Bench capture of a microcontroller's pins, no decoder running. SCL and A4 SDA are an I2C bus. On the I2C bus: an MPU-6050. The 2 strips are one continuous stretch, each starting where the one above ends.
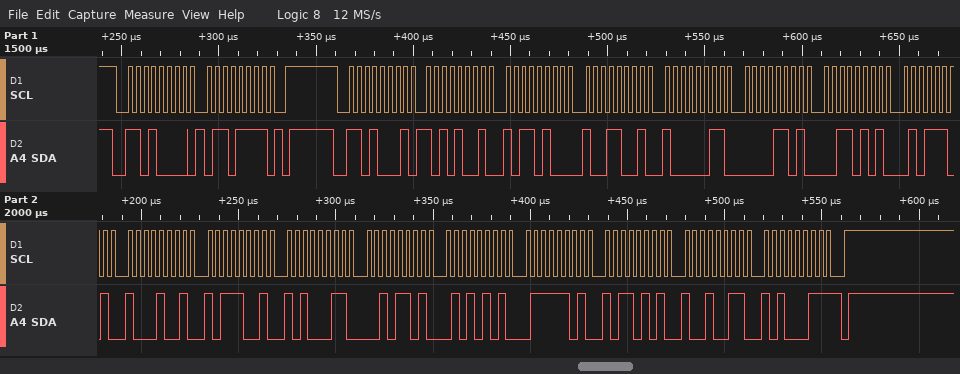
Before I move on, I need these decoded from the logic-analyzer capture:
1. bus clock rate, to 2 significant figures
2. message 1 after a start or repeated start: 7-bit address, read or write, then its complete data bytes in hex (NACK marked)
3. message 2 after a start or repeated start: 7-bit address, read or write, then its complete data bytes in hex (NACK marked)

250 kHz
0x68 write: 6F
0x68 read: A9 B4 99 83 0D 35 5D 89 B9 A3 2D 55 7D B5 93 A3 NACK
